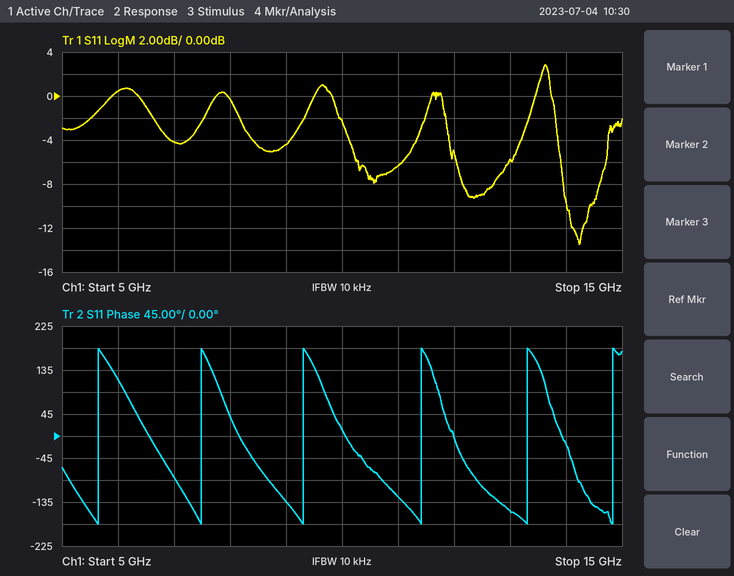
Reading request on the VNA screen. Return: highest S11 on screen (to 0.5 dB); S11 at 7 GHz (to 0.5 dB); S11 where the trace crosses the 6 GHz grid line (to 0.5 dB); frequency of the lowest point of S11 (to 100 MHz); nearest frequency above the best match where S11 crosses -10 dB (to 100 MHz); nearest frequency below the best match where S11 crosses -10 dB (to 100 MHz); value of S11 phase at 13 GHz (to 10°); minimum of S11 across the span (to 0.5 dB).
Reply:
3.0 dB
-4.0 dB
0.5 dB
14.2 GHz
14.4 GHz
14.0 GHz
-150°
-13.5 dB
